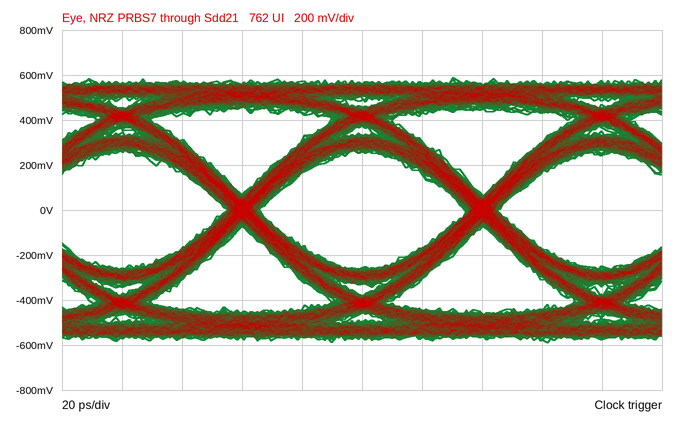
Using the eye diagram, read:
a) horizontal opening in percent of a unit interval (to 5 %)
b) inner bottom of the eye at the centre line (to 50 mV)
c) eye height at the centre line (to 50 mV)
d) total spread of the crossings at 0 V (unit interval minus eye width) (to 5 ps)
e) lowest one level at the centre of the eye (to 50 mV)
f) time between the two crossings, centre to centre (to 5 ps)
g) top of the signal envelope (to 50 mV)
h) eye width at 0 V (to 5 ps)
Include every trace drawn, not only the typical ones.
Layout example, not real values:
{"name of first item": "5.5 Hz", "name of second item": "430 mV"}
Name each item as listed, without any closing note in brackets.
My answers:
{"horizontal opening in percent of a unit interval": "85 %", "inner bottom of the eye at the centre line": "-250 mV", "eye height at the centre line": "500 mV", "total spread of the crossings at 0 V (unit interval minus eye width)": "10 ps", "lowest one level at the centre of the eye": "250 mV", "time between the two crossings, centre to centre": "80 ps", "top of the signal envelope": "600 mV", "eye width at 0 V": "70 ps"}
